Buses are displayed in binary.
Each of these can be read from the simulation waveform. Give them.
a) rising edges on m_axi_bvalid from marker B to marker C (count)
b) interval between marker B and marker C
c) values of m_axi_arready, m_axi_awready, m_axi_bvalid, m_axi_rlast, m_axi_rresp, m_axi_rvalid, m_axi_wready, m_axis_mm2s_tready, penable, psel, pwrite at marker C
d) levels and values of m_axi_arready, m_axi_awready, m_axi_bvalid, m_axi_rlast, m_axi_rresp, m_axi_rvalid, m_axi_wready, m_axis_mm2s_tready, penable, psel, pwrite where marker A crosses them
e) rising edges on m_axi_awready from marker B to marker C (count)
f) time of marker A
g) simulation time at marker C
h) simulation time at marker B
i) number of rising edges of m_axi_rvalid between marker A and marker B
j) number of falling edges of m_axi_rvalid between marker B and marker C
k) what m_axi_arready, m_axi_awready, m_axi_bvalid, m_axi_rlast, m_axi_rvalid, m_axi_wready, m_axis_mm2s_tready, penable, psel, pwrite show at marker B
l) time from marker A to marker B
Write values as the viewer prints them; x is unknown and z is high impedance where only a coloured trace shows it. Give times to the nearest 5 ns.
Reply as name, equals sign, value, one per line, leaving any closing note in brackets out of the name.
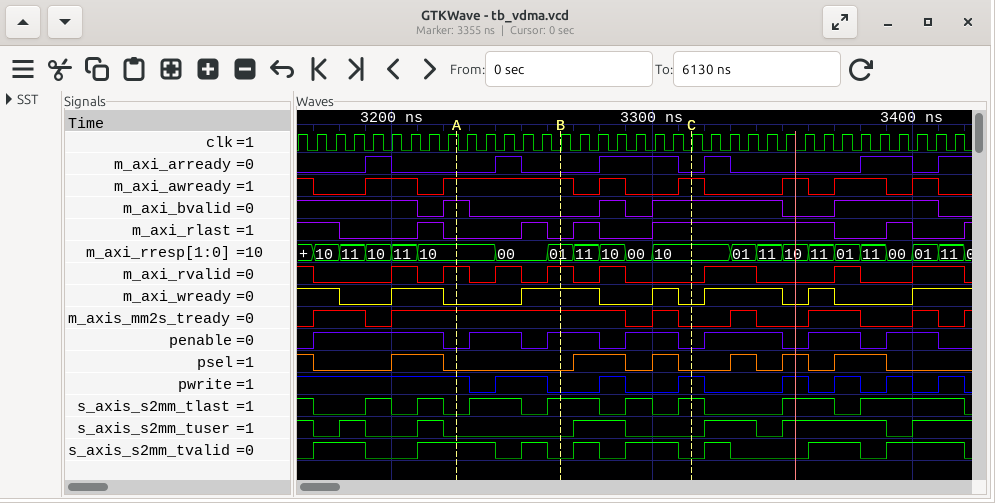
rising edges on m_axi_bvalid from marker B to marker C = 2
interval between marker B and marker C = 50 ns
values of m_axi_arready, m_axi_awready, m_axi_bvalid, m_axi_rlast, m_axi_rresp, m_axi_rvalid, m_axi_wready, m_axis_mm2s_tready, penable, psel, pwrite at marker C = m_axi_arready=0, m_axi_awready=1, m_axi_bvalid=1, m_axi_rlast=1, m_axi_rresp=10, m_axi_rvalid=0, m_axi_wready=0, m_axis_mm2s_tready=0, penable=0, psel=0, pwrite=1
levels and values of m_axi_arready, m_axi_awready, m_axi_bvalid, m_axi_rlast, m_axi_rresp, m_axi_rvalid, m_axi_wready, m_axis_mm2s_tready, penable, psel, pwrite where marker A crosses them = m_axi_arready=0, m_axi_awready=1, m_axi_bvalid=1, m_axi_rlast=0, m_axi_rresp=10, m_axi_rvalid=1, m_axi_wready=0, m_axis_mm2s_tready=1, penable=0, psel=0, pwrite=1
rising edges on m_axi_awready from marker B to marker C = 2
time of marker A = 3225 ns
simulation time at marker C = 3315 ns
simulation time at marker B = 3265 ns
number of rising edges of m_axi_rvalid between marker A and marker B = 2
number of falling edges of m_axi_rvalid between marker B and marker C = 2
what m_axi_arready, m_axi_awready, m_axi_bvalid, m_axi_rlast, m_axi_rvalid, m_axi_wready, m_axis_mm2s_tready, penable, psel, pwrite show at marker B = m_axi_arready=0, m_axi_awready=1, m_axi_bvalid=0, m_axi_rlast=0, m_axi_rvalid=1, m_axi_wready=1, m_axis_mm2s_tready=1, penable=1, psel=0, pwrite=0
time from marker A to marker B = 40 ns
